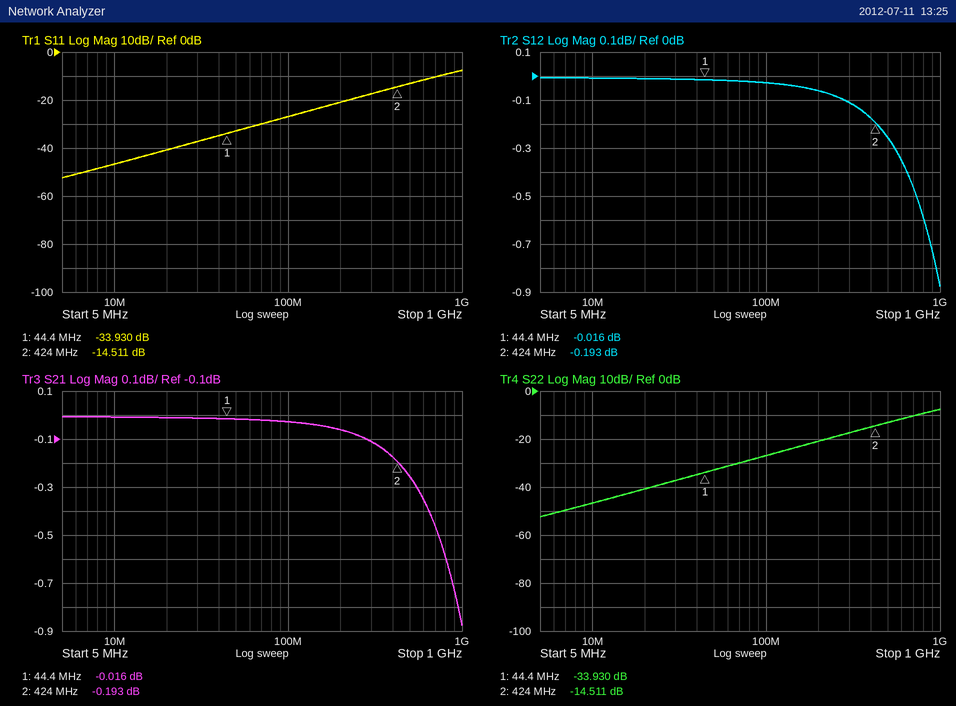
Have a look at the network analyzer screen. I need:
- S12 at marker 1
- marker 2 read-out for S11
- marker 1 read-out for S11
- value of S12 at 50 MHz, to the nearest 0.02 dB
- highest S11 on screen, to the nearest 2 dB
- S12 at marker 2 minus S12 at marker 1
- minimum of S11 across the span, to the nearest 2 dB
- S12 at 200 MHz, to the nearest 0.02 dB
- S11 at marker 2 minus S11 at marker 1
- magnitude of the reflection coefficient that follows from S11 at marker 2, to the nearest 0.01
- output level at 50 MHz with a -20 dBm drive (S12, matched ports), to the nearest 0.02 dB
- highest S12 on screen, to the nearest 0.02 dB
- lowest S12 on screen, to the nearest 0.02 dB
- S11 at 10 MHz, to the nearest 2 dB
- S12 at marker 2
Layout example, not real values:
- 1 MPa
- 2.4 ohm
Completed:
- -0.016 dB
- -14.511 dB
- -33.930 dB
- -0.02 dB
- -8 dB
- -0.177 dB
- -52 dB
- -0.06 dB
- 19.419 dB
- 0.19
- -20.02 dBm
- 0.00 dB
- -0.88 dB
- -46 dB
- -0.193 dB
